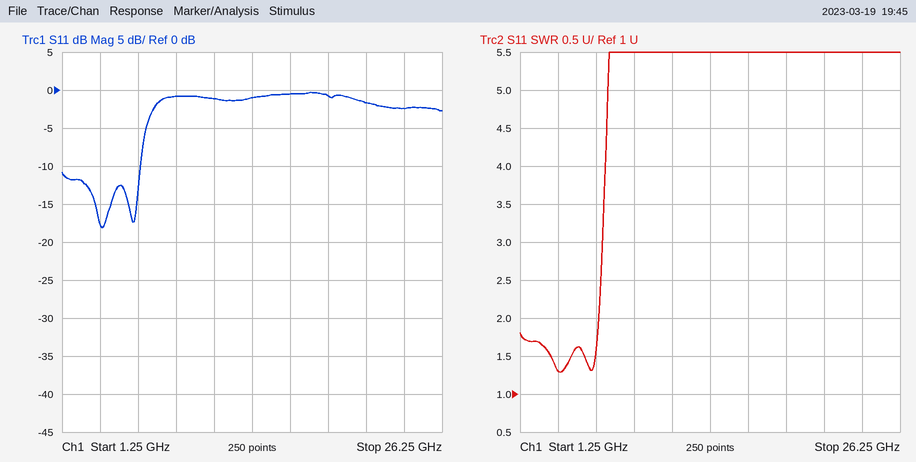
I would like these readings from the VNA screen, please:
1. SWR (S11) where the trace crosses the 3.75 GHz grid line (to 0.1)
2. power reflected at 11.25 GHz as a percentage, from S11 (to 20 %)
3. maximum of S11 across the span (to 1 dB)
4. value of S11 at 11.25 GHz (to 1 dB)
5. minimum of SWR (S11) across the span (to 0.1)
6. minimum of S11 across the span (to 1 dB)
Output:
1.3
80 %
0 dB
-1 dB
1.3
-18 dB
